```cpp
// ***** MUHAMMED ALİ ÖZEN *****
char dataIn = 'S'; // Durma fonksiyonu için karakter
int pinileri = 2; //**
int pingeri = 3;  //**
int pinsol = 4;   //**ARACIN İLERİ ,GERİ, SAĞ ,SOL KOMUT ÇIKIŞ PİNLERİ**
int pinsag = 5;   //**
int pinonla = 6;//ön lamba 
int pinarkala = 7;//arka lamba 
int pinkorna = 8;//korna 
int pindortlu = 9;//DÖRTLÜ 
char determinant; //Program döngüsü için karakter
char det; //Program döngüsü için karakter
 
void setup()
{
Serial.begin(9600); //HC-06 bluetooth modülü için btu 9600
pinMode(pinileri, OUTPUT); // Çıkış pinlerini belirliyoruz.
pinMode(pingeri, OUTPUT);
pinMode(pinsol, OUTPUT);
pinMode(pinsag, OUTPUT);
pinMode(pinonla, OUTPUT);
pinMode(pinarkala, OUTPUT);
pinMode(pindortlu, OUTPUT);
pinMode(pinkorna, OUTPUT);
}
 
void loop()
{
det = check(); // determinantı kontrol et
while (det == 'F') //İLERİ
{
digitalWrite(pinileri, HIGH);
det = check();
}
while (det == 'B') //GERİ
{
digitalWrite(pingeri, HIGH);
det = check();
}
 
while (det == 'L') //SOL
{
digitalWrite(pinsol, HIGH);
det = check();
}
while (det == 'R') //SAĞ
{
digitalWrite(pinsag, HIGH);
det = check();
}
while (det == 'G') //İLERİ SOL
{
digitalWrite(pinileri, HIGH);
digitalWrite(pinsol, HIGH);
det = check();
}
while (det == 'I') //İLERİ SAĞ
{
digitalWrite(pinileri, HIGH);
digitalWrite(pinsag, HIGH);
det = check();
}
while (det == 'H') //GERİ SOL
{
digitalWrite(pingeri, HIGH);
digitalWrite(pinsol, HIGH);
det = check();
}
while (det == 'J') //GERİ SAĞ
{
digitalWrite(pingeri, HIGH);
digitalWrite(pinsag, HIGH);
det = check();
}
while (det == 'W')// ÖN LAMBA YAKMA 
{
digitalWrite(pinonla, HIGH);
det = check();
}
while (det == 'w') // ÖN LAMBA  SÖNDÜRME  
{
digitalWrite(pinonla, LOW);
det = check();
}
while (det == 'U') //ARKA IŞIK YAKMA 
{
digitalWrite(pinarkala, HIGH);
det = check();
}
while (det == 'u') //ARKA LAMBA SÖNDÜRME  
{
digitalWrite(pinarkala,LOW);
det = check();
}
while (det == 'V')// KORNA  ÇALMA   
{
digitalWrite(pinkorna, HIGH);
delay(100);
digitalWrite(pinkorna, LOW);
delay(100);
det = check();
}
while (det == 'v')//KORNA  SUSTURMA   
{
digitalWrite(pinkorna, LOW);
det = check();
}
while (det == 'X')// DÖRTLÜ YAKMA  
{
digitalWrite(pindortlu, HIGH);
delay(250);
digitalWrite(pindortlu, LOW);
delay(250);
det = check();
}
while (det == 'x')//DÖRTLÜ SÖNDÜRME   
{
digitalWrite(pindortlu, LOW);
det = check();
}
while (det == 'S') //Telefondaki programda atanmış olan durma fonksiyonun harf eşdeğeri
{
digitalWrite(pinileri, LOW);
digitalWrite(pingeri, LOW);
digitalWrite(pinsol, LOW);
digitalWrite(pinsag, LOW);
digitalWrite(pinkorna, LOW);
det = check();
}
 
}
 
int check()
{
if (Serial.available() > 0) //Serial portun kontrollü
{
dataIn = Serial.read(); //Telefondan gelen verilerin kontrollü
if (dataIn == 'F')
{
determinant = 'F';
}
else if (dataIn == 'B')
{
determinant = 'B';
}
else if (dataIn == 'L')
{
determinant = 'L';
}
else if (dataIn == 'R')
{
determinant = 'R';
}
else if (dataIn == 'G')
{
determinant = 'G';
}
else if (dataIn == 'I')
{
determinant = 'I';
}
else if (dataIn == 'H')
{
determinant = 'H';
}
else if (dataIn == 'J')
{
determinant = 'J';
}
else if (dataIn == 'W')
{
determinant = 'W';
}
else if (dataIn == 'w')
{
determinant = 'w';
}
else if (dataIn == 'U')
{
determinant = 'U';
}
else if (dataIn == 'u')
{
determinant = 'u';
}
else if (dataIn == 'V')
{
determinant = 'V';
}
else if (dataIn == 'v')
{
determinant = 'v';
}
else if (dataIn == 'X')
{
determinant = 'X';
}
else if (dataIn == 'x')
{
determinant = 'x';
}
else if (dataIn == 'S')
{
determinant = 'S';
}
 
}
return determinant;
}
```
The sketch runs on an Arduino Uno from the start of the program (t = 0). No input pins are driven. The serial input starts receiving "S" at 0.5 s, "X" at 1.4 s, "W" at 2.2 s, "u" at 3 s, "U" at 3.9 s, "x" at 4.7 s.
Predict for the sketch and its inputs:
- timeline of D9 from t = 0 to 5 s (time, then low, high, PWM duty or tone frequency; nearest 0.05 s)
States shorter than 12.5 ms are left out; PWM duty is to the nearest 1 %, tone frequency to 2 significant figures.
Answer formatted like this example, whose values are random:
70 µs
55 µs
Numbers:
0 s low; 1.4 s high; 1.65 s low; 1.9 s high; 2.15 s low
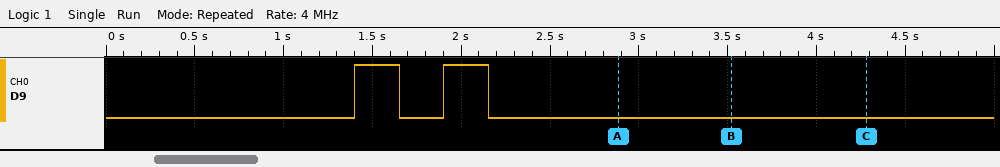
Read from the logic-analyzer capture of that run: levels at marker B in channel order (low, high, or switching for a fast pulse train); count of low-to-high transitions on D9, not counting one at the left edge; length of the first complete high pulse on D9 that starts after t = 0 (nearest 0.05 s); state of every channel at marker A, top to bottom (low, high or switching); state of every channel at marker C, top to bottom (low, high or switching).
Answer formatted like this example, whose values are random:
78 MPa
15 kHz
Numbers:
D9 low
2
0.25 s
D9 low
D9 low
